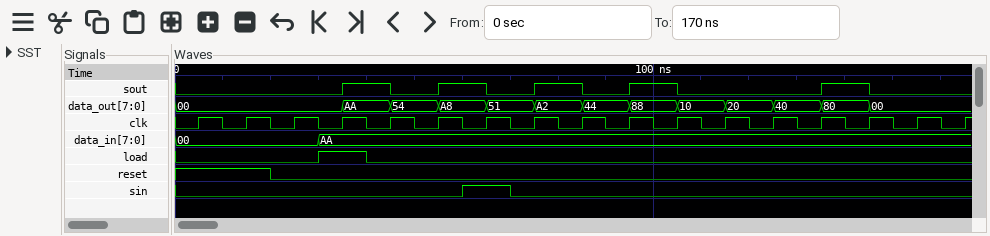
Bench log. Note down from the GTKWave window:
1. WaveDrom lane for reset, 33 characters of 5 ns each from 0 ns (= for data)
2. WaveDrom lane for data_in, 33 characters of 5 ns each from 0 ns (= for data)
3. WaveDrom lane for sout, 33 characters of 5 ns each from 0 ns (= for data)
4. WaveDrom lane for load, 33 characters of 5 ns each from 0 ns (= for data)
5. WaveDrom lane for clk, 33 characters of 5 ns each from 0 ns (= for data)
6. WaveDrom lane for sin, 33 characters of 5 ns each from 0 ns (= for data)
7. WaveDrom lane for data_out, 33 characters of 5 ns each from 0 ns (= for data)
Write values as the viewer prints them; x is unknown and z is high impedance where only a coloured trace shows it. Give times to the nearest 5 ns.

{name: 'reset', wave: '1...0............................'}
{name: 'data_in', wave: '=.....=..........................', data: '00 AA'}
{name: 'sout', wave: '0......1.0.1.0.1.0.1.0.....1.0...'}
{name: 'load', wave: '0.....1.0........................'}
{name: 'clk', wave: '010101010101010101010101010101010'}
{name: 'sin', wave: '0...........1.0..................'}
{name: 'data_out', wave: '=......=.=.=.=.=.=.=.=.=.=.=.=...', data: '00 AA 54 A8 51 A2 44 88 10 20 40 80 00'}
